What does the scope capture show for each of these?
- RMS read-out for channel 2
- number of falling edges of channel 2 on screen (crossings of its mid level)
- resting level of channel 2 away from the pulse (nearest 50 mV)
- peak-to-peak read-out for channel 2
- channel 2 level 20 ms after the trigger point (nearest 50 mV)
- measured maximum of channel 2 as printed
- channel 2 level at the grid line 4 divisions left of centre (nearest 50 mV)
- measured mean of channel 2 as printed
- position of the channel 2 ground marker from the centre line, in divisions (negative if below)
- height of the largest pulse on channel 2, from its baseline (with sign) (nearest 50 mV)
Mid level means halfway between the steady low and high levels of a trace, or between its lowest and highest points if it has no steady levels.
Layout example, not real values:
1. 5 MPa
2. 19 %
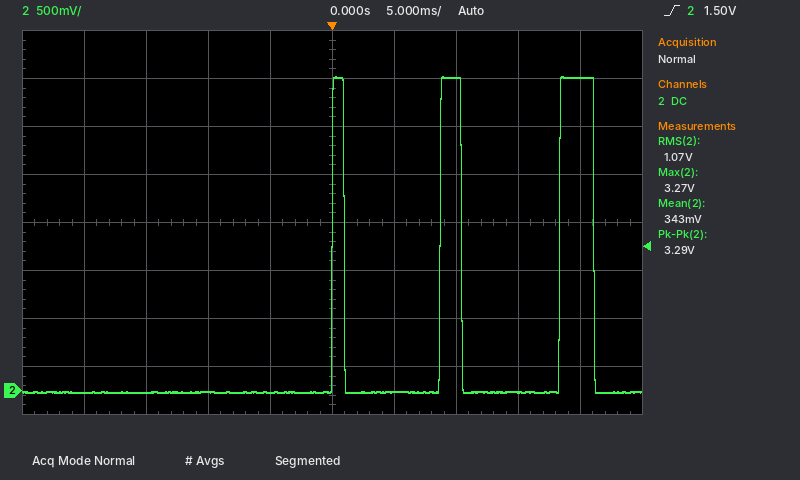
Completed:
1. 1.07 V
2. 3
3. 0 mV
4. 3.29 V
5. 3.25 V
6. 3.27 V
7. 0 mV
8. 343 mV
9. -3.5 div
10. +3.30 V
